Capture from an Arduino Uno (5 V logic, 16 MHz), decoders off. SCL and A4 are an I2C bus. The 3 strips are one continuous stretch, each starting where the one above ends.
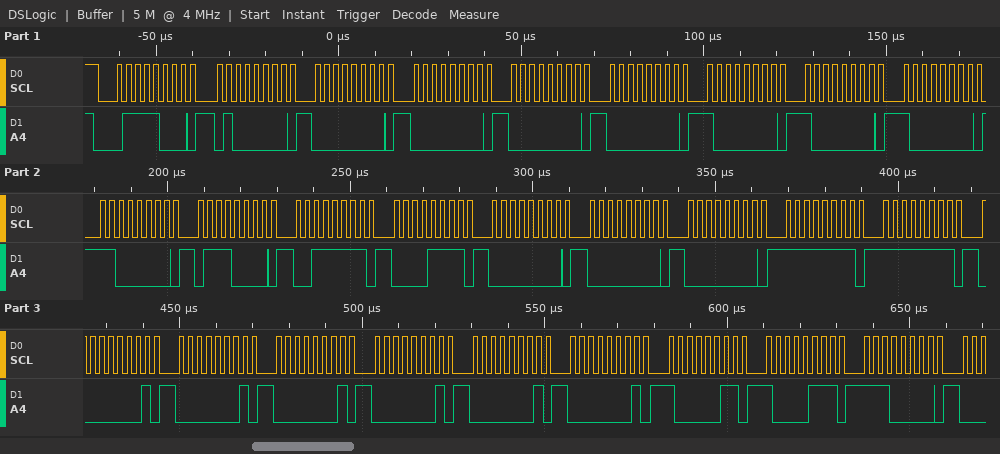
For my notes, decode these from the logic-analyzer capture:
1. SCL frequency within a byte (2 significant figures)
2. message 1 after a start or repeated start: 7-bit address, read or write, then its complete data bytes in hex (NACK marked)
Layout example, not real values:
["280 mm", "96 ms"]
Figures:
["400 kHz", "0x3C write: 40 00 00 00 00 80 80 80 C0 70 3F 0F 00 00 00 FF FF 01 01 01 01 01 01 83 87 E0"]
